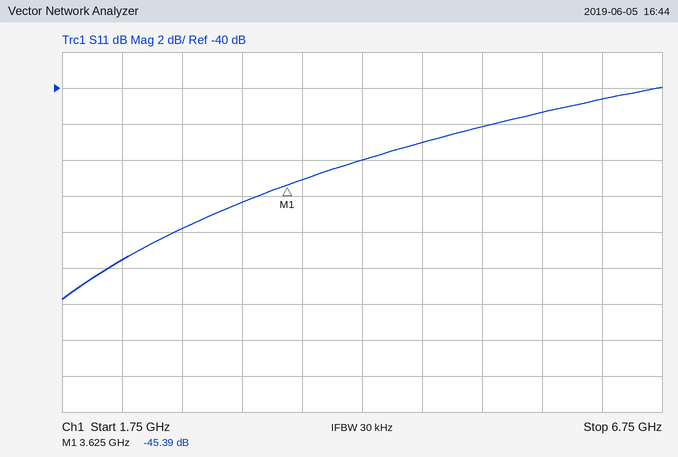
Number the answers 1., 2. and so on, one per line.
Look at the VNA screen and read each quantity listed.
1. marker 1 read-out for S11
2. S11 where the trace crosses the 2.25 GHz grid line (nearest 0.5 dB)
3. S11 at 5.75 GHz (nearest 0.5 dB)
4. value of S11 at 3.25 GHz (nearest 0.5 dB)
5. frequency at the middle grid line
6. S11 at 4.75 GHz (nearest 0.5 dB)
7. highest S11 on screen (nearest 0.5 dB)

1. -45.39 dB
2. -49.5 dB
3. -41.5 dB
4. -46.5 dB
5. 4.25 GHz
6. -43.0 dB
7. -40.0 dB
